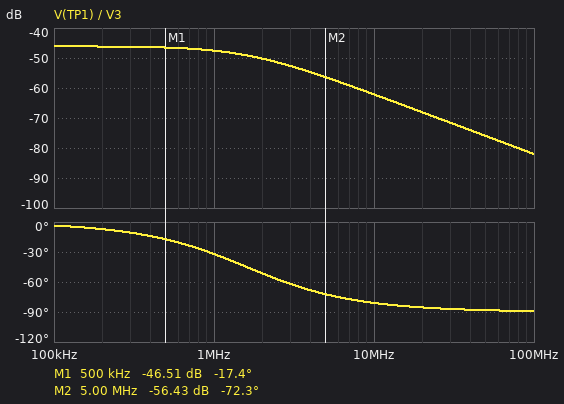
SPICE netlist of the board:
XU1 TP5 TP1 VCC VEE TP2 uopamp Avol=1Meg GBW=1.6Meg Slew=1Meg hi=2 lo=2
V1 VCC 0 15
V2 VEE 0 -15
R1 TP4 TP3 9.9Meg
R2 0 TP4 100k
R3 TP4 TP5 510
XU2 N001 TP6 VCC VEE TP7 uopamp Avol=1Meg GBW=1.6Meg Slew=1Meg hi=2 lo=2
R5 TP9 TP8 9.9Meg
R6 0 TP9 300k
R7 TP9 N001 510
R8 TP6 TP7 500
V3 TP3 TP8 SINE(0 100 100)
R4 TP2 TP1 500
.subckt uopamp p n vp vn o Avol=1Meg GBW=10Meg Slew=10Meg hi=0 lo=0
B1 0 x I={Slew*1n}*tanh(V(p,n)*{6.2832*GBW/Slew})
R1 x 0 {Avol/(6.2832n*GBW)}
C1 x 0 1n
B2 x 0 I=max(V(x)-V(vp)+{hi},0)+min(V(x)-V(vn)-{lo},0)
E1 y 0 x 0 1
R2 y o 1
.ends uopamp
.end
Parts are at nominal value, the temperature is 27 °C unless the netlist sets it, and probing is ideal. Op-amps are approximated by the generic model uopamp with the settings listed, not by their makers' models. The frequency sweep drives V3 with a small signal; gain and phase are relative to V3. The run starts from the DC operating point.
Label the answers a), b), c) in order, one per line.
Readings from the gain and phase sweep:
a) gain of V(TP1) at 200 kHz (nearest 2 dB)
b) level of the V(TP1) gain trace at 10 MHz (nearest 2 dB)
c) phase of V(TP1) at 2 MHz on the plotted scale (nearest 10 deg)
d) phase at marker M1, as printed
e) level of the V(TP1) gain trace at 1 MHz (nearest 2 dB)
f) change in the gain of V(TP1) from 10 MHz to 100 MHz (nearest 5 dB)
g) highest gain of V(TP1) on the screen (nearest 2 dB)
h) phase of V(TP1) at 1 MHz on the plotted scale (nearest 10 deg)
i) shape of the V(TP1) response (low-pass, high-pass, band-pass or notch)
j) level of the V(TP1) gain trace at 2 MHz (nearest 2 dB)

a) -46 dB
b) -62 dB
c) -50 deg
d) -17.4 deg
e) -48 dB
f) -20 dB
g) -46 dB
h) -30 deg
i) low-pass
j) -50 dB
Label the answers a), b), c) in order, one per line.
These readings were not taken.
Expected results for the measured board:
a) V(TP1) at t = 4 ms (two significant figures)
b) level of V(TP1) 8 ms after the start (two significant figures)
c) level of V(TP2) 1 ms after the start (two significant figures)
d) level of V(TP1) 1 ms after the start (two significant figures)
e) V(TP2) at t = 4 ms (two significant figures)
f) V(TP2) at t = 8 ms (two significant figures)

a) 290 mV
b) -470 mV
c) 290 mV
d) 290 mV
e) 290 mV
f) -470 mV
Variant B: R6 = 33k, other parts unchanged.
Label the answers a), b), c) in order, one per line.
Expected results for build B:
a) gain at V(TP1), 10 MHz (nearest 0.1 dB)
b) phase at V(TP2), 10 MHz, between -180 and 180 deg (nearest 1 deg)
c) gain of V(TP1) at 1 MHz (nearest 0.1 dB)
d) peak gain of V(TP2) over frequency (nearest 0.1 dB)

a) -62.0 dB
b) -81 deg
c) -47.4 dB
d) -46.0 dB
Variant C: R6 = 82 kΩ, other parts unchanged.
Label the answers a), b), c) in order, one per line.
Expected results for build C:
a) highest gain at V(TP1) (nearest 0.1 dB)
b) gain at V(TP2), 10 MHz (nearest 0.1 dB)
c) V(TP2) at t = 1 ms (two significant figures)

a) -46.0 dB
b) -62.0 dB
c) 290 mV
